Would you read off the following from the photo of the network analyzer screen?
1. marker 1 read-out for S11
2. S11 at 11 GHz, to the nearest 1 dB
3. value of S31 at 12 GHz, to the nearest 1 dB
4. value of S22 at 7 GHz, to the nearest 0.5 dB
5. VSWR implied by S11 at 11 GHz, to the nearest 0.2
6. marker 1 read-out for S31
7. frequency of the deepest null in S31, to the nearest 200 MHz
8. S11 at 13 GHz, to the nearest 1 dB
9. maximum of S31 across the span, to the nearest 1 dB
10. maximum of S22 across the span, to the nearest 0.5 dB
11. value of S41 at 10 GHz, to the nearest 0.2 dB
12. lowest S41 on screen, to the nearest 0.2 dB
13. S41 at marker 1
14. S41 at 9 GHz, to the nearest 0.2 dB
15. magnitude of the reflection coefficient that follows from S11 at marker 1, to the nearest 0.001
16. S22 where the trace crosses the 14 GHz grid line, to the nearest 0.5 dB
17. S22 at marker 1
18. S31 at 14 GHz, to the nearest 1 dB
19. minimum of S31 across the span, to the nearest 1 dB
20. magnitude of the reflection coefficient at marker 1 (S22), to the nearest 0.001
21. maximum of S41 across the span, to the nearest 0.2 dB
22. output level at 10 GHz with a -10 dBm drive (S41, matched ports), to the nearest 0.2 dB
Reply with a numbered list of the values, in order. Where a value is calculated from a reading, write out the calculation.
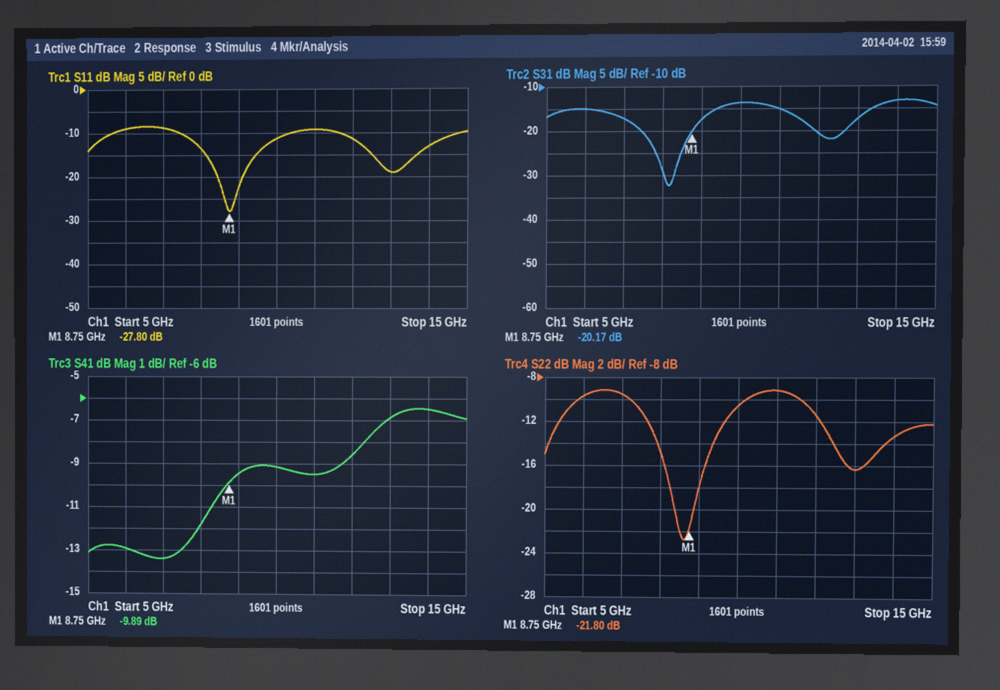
1. -27.80 dB
2. -9 dB
3. -21 dB
4. -9.5 dB
5. |Γ| = 10^(-9/20) = 0.3548; VSWR = (1 + 0.3548)/(1 − 0.3548) ≈ 2.10, so 2.0 to the nearest 0.2
6. -20.17 dB
7. 8.2 GHz
8. -19 dB
9. -13 dB
10. -9.0 dB
11. -9.2 dB
12. -13.4 dB
13. -9.89 dB
14. -9.4 dB
15. 10^(-27.8/20) ≈ 0.041
16. -13.5 dB
17. -21.80 dB
18. -13 dB
19. -32 dB
20. 10^(-21.8/20) ≈ 0.081
21. -6.4 dB
22. -10 dBm + (-9.2 dB) = -19.2 dBm
